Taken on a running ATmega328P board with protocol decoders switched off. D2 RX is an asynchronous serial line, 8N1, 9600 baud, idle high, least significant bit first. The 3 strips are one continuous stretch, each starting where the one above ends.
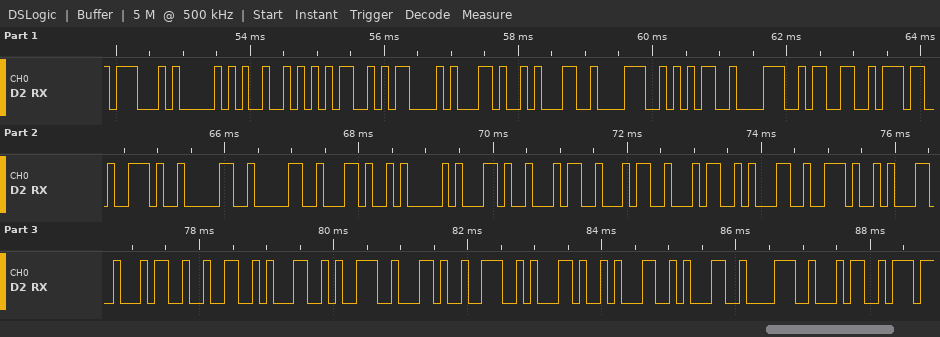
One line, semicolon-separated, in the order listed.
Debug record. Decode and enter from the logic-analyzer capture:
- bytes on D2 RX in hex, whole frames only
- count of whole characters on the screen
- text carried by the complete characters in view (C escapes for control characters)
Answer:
47 50 52 4D 43 2C 31 38 35 38 33 37 2E 30 30 2C 41 2C 34 34 34 31 2E 31 34 32 31 39 2C 4E 2C 31 31 38 34; 35; "GPRMC,185837.00,A,4441.14219,N,1184"
